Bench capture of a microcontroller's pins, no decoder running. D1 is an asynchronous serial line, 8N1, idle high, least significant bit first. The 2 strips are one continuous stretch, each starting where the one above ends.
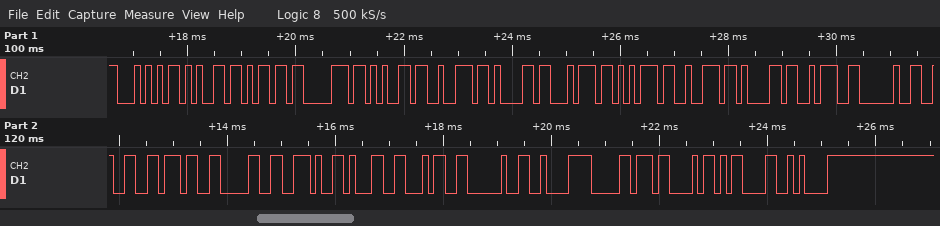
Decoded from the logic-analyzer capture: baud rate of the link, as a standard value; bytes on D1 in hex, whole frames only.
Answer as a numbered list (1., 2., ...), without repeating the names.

1. 9600 baud
2. 54 65 6D 70 65 72 61 74 75 72 61 3A 20 32 37 30 2E 31 34 20 C2 B0 43 0D 0A
